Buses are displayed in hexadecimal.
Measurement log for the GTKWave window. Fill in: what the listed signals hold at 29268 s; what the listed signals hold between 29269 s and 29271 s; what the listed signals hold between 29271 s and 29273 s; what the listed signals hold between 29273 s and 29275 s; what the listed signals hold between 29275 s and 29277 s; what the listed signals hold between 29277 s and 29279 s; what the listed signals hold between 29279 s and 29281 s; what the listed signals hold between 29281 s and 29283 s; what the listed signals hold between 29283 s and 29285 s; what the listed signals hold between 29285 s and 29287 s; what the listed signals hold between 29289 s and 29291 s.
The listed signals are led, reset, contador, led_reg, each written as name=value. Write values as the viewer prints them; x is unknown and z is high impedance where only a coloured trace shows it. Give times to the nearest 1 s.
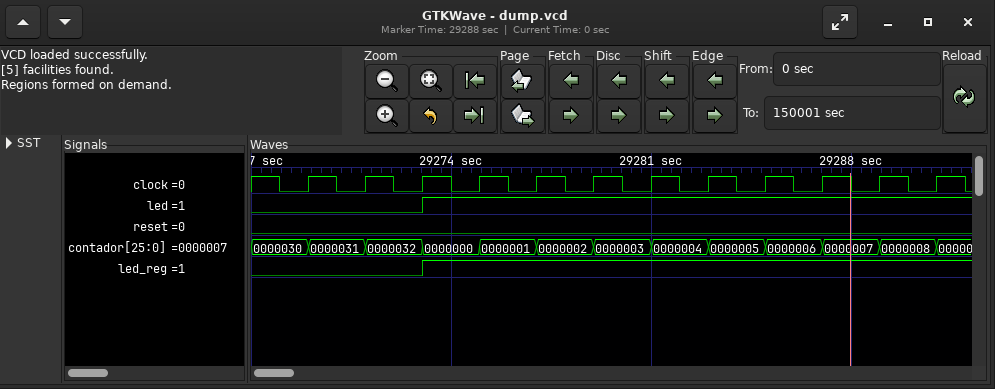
led=0, reset=0, contador=0000030, led_reg=0
led=0, reset=0, contador=0000031, led_reg=0
led=0, reset=0, contador=0000032, led_reg=0
led=1, reset=0, contador=0000000, led_reg=1
led=1, reset=0, contador=0000001, led_reg=1
led=1, reset=0, contador=0000002, led_reg=1
led=1, reset=0, contador=0000003, led_reg=1
led=1, reset=0, contador=0000004, led_reg=1
led=1, reset=0, contador=0000005, led_reg=1
led=1, reset=0, contador=0000006, led_reg=1
led=1, reset=0, contador=0000008, led_reg=1
